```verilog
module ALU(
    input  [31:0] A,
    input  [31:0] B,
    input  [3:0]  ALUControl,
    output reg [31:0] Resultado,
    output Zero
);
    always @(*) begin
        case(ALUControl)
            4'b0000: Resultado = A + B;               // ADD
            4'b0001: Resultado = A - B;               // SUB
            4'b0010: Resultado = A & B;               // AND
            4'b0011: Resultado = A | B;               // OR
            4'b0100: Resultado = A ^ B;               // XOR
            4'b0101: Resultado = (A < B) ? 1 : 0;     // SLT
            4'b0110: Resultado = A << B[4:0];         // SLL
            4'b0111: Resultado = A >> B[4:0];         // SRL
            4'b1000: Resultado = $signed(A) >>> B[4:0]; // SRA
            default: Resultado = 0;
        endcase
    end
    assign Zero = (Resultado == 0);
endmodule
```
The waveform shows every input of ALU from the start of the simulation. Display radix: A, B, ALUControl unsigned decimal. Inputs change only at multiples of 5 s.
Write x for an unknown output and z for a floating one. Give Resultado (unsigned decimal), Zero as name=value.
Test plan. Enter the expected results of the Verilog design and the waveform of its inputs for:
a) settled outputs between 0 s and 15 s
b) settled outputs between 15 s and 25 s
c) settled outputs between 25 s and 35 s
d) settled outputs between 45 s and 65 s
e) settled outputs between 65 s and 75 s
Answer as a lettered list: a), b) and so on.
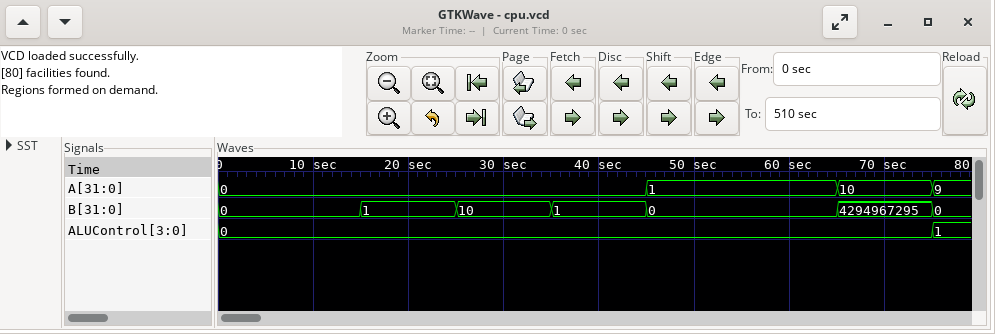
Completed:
a) Resultado=0, Zero=1
b) Resultado=1, Zero=0
c) Resultado=10, Zero=0
d) Resultado=1, Zero=0
e) Resultado=9, Zero=0
